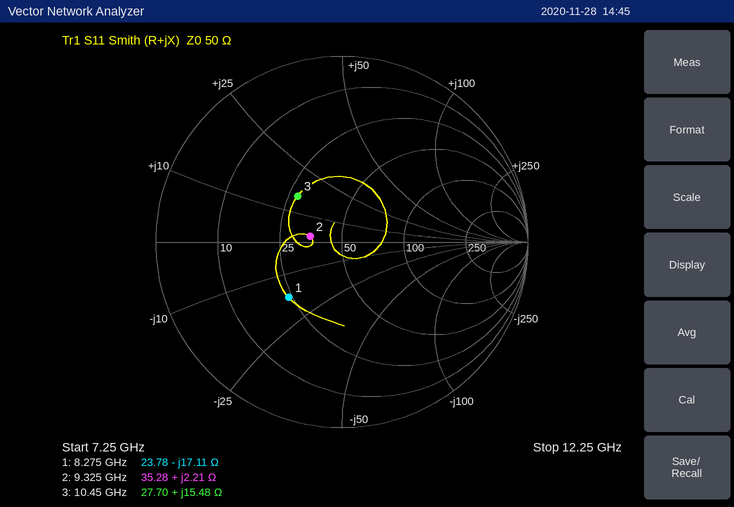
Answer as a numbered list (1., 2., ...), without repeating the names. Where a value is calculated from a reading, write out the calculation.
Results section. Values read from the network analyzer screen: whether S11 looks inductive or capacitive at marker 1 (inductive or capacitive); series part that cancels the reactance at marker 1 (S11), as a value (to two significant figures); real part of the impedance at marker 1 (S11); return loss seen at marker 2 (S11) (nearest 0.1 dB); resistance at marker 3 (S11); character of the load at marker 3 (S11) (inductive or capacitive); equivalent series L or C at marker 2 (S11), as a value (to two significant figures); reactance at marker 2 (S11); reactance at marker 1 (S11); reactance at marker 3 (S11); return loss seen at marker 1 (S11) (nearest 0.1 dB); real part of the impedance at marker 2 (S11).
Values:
1. capacitive
2. L = 17.11 Ω/(2π × 8.275 GHz) ≈ 329 pH, so 330 pH to two significant figures
3. 23.78 Ω
4. 15.2 dB
5. 27.70 Ω
6. inductive
7. L = 2.21 Ω/(2π × 9.325 GHz) ≈ 38 pH
8. +2.21 Ω
9. -17.11 Ω
10. +15.48 Ω
11. 7.7 dB
12. 35.28 Ω
